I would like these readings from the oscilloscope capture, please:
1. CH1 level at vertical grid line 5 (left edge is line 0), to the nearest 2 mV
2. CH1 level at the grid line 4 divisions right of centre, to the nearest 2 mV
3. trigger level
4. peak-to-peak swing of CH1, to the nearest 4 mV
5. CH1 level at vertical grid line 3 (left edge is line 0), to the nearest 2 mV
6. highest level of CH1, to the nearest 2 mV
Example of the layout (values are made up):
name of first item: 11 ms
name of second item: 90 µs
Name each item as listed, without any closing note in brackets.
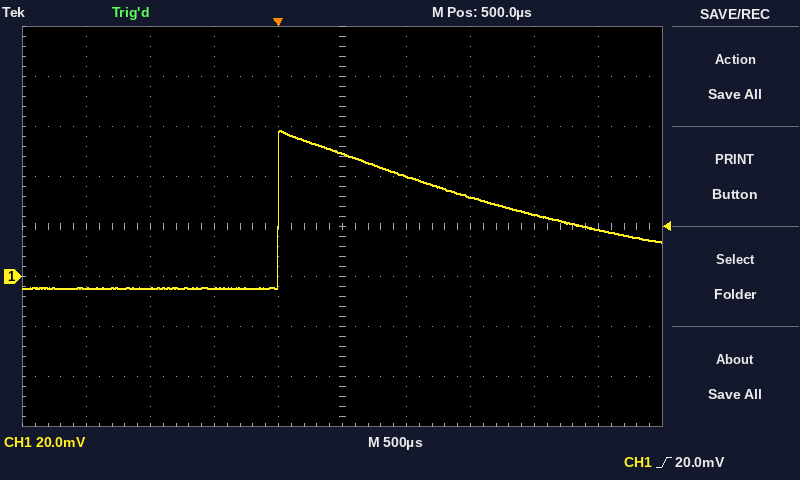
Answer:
CH1 level at vertical grid line 5 (left edge is line 0), to the nearest 2 mV: 50 mV
CH1 level at the grid line 4 divisions right of centre, to the nearest 2 mV: 18 mV
trigger level: 20.0 mV
peak-to-peak swing of CH1, to the nearest 4 mV: 64 mV
CH1 level at vertical grid line 3 (left edge is line 0), to the nearest 2 mV: -4 mV
highest level of CH1, to the nearest 2 mV: 58 mV
